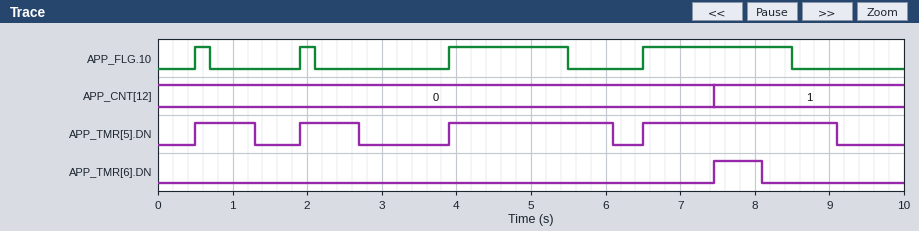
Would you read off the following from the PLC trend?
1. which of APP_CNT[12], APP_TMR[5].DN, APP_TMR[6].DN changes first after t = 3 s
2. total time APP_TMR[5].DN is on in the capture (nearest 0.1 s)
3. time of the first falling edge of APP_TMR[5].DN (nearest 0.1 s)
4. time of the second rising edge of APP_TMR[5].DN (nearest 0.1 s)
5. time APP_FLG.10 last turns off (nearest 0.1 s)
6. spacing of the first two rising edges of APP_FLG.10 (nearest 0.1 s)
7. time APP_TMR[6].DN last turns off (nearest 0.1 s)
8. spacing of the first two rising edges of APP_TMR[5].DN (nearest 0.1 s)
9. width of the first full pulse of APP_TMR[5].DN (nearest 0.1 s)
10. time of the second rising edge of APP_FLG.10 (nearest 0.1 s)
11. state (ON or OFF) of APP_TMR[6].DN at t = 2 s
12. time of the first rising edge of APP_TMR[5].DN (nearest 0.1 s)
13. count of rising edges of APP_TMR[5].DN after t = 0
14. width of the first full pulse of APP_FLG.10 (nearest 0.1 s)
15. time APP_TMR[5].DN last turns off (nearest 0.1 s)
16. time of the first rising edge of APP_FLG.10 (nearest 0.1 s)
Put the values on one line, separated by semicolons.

APP_TMR[5].DN; 6.4 s; 1.3 s; 1.9 s; 8.5 s; 1.4 s; 8.1 s; 1.4 s; 0.8 s; 1.9 s; OFF; 0.5 s; 4; 0.2 s; 9.1 s; 0.5 s
